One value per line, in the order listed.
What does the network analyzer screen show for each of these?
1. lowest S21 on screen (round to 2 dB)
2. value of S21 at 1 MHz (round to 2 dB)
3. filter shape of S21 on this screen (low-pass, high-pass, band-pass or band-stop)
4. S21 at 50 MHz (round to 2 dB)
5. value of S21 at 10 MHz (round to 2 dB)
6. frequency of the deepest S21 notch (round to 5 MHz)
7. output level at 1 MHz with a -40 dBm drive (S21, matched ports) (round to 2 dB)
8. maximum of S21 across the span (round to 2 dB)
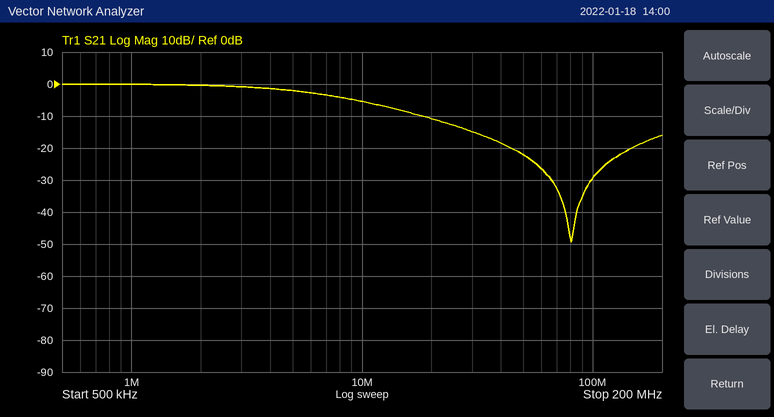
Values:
-50 dB
0 dB
low-pass
-22 dB
-6 dB
80 MHz
-40 dBm
0 dB
